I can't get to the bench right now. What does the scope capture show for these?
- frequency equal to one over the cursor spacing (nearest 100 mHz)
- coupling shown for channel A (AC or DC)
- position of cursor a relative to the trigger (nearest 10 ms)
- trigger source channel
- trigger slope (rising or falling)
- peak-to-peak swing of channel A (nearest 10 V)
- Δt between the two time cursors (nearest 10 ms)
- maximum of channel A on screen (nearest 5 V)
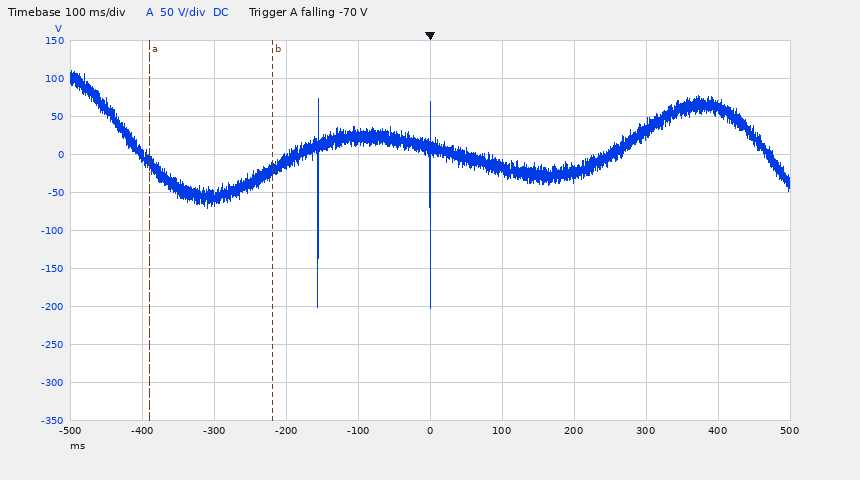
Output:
5.9 Hz
DC
-390 ms
channel A
falling
310 V
170 ms
110 V
